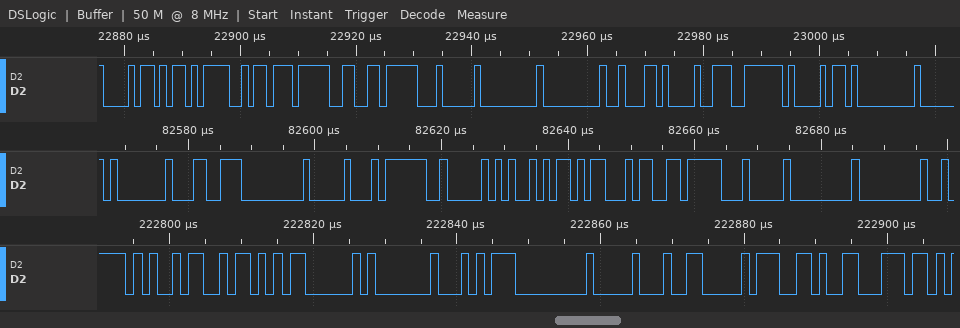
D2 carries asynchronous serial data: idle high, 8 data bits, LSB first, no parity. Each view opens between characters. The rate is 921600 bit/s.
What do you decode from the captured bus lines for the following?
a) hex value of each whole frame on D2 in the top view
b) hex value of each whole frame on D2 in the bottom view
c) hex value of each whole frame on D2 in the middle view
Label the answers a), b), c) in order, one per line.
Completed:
a) 68, EB, DA, 9F, F6, 04, 00, 00, 62, C8, 7E, 68, 00
b) A5, 5A, 03, 01, D4, 00, 10, 06, 67, C6
c) 01, CC, 00, 10, 3F, 50, 6A, A3, F6, 04, 00, 00
